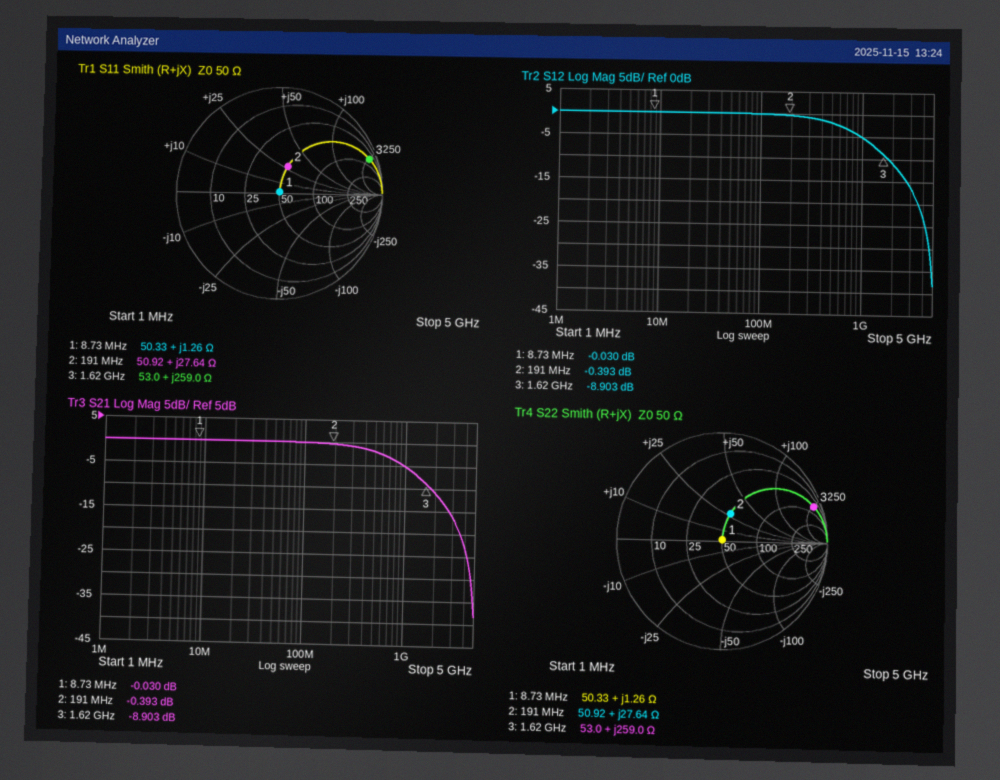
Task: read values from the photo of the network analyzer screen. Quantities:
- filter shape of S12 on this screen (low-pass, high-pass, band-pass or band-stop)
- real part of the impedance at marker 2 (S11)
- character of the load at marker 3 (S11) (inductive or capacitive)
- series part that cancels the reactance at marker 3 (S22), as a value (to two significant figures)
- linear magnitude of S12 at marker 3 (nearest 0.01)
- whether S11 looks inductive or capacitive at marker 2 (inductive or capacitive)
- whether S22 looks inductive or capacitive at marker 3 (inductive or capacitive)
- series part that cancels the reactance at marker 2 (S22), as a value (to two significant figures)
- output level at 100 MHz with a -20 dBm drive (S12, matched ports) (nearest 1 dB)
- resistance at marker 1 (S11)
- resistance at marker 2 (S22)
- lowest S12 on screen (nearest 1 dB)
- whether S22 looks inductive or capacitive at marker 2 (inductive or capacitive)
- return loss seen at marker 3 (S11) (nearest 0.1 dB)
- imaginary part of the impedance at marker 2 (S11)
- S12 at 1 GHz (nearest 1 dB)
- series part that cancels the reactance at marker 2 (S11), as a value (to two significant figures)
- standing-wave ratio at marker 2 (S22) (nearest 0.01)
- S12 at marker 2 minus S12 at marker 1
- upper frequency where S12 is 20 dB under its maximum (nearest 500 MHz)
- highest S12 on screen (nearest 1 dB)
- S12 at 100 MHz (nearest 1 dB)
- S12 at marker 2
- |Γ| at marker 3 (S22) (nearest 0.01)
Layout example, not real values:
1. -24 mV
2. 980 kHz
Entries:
1. low-pass
2. 50.92 Ω
3. inductive
4. 380 fF
5. 0.36
6. inductive
7. inductive
8. 30 pF
9. -20 dBm
10. 50.33 Ω
11. 50.92 Ω
12. -38 dB
13. inductive
14. 0.6 dB
15. +27.64 Ω
16. -5 dB
17. 30 pF
18. 1.72
19. -0.363 dB
20. 3.5 GHz
21. 0 dB
22. 0 dB
23. -0.393 dB
24. 0.93
